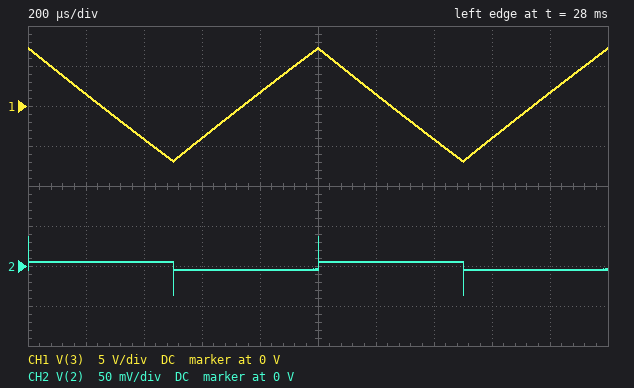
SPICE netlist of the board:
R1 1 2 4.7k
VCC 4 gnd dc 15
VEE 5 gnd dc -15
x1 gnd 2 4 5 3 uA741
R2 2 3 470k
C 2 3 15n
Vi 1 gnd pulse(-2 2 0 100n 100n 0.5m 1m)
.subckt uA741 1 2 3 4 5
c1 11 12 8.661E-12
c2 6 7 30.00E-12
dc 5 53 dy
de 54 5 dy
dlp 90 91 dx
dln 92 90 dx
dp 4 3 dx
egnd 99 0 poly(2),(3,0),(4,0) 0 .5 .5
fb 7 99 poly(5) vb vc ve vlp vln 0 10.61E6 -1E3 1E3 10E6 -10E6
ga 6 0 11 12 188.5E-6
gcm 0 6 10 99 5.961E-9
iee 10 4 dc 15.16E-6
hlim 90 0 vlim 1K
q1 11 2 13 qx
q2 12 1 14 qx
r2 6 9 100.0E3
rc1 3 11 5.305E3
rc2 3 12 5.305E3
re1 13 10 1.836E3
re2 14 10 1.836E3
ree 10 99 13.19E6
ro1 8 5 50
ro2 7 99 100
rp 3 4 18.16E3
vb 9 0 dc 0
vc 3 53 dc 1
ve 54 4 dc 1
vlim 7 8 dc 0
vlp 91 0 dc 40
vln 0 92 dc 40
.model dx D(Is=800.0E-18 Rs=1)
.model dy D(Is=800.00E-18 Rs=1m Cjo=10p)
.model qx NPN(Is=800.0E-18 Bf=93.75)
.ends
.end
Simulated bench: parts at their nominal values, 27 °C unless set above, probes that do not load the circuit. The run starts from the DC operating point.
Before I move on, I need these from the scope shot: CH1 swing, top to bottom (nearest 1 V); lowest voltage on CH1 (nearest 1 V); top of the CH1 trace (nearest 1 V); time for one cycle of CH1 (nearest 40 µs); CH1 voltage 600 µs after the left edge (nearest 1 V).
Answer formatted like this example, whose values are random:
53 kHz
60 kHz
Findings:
14 V
-7 V
7 V
1.00 ms
-4 V
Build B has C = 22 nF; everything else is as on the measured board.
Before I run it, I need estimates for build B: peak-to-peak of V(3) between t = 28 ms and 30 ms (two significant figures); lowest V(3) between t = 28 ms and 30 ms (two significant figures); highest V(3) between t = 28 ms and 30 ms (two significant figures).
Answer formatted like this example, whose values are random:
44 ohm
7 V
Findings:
9.8 V
-4.2 V
5.6 V
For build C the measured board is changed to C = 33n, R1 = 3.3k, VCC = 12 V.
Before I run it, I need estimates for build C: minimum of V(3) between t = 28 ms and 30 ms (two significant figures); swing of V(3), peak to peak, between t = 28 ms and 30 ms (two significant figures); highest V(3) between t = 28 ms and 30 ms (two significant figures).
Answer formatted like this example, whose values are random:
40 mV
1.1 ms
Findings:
-3.4 V
9.4 V
6.0 V
